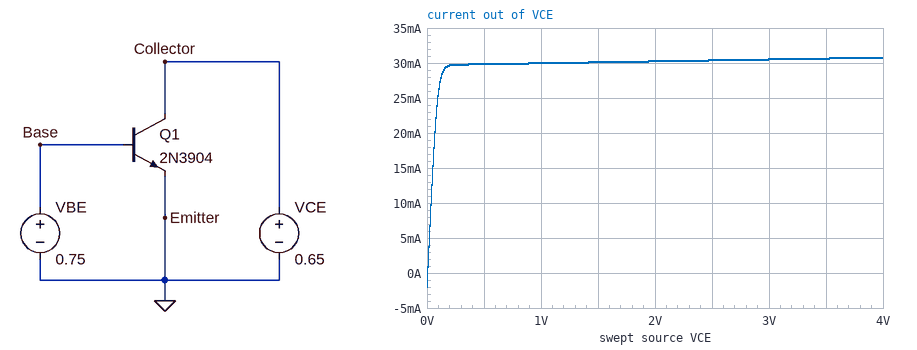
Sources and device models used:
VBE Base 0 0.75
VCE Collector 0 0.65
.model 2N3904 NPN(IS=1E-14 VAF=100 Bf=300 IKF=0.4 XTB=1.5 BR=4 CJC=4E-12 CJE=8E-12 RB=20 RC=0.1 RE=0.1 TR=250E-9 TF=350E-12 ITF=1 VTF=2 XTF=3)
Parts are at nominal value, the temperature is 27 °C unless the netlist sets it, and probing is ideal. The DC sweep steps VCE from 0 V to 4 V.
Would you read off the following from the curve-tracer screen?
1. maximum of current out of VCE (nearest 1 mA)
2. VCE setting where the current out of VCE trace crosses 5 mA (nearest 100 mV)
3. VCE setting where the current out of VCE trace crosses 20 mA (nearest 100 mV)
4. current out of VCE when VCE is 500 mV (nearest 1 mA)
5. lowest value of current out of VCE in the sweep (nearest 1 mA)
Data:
31 mA
0 V
100 mV
30 mA
-2 mA
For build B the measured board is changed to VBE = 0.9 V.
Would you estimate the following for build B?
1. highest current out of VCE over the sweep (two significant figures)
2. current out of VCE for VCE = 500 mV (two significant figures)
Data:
350 mA
340 mA
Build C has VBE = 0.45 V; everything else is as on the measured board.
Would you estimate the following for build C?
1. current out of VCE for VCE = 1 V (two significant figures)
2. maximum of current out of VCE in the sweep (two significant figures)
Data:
360 nA
370 nA
